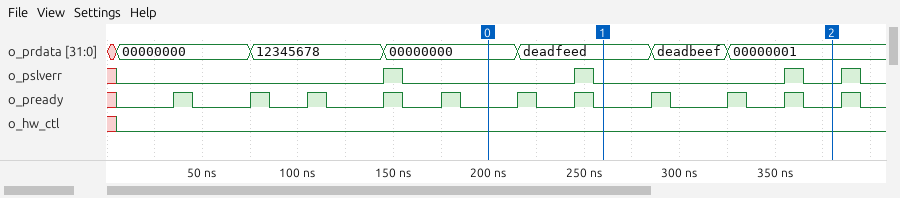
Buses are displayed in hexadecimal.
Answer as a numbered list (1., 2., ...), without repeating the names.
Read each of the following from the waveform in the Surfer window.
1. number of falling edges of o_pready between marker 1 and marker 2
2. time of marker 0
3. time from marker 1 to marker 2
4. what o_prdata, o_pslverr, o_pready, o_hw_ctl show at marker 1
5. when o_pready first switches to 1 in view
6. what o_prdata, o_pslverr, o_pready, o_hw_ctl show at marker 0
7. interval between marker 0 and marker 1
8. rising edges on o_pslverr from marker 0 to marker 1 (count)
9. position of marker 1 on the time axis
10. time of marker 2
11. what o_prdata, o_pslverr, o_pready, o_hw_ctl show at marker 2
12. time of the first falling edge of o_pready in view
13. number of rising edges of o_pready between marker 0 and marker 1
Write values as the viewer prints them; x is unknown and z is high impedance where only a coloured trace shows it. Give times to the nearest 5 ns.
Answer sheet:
1. 3
2. 200 ns
3. 120 ns
4. o_prdata=deadfeed, o_pslverr=0, o_pready=0, o_hw_ctl=0
5. 35 ns
6. o_prdata=00000000, o_pslverr=0, o_pready=0, o_hw_ctl=0
7. 60 ns
8. 1
9. 260 ns
10. 380 ns
11. o_prdata=00000001, o_pslverr=0, o_pready=0, o_hw_ctl=0
12. 45 ns
13. 2
